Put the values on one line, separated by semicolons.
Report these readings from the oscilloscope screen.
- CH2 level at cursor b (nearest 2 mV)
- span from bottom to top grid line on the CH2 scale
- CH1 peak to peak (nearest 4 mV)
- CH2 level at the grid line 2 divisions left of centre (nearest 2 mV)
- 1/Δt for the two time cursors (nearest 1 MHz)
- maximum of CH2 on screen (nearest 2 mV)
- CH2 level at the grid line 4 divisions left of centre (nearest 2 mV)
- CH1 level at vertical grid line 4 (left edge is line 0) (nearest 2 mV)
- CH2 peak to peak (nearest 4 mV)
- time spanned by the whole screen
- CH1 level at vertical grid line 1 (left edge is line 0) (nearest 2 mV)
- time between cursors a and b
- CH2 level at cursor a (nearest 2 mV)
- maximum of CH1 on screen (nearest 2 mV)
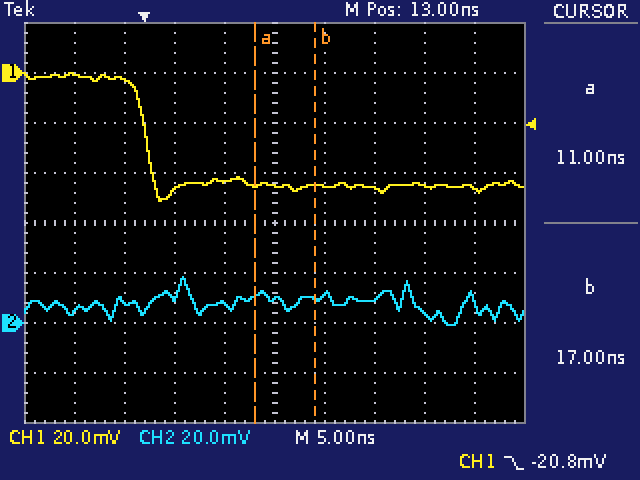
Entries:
10 mV; 160 mV; 52 mV; 10 mV; 167 MHz; 18 mV; 4 mV; -44 mV; 20 mV; 50 ns; 0 mV; 6.0 ns; 10 mV; 0 mV
